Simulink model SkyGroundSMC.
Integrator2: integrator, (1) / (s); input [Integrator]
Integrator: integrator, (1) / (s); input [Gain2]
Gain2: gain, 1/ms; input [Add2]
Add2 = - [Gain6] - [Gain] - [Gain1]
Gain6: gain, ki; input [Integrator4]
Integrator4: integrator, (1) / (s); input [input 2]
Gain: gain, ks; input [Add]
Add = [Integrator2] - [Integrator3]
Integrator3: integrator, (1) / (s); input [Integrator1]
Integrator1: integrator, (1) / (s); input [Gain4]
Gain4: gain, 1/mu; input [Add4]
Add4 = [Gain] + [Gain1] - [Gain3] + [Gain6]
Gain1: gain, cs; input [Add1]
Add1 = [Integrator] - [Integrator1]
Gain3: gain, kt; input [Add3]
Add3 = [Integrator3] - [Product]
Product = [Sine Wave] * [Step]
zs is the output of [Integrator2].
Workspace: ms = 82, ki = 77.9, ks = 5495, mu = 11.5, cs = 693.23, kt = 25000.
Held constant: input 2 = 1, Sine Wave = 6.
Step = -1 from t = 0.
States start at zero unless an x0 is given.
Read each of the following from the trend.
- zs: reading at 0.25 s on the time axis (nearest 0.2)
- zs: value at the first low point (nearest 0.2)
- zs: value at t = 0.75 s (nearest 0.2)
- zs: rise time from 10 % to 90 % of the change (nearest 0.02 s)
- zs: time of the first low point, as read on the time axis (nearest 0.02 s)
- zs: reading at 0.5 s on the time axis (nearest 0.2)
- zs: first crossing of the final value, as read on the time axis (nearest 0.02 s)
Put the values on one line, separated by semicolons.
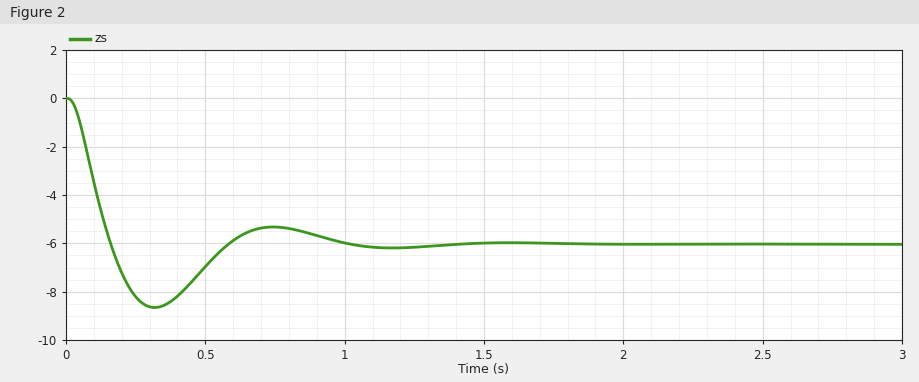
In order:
-8.2; -8.6; -5.4; 0.10 s; 0.32 s; -7.0; 0.16 s
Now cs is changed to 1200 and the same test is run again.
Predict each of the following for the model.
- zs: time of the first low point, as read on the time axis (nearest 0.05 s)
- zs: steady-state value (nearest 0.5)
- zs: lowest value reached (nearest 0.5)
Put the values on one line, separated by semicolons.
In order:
0.25 s; -6.0; -8.5
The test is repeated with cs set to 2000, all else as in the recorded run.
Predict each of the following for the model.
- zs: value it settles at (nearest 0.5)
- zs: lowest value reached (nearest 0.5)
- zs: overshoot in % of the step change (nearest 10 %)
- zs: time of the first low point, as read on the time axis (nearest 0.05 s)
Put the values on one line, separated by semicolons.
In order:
-6.0; -9.0; 40 %; 0.20 s
